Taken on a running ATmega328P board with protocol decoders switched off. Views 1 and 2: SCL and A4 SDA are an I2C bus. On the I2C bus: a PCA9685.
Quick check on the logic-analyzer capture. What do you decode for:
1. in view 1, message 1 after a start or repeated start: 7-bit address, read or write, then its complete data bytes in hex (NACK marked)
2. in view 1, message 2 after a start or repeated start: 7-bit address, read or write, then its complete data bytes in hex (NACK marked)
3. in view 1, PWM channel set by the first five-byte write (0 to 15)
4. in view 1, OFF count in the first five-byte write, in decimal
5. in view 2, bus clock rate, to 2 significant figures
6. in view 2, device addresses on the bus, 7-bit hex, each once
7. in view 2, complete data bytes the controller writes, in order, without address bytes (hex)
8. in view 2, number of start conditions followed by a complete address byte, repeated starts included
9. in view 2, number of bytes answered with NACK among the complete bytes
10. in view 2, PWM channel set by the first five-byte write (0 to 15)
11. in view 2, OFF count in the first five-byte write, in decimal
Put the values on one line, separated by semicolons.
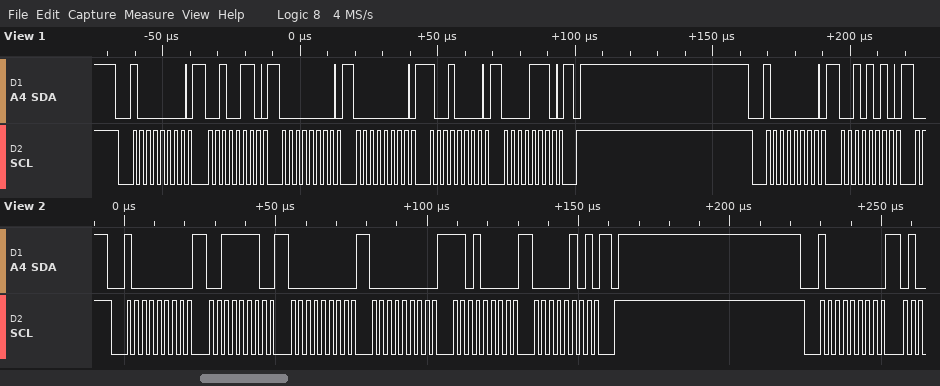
0x40 write: 26 00 00 90 0E; 0x40 write: 2A; 8; 3728; 400 kHz; 0x40; 3E 00 00 D0 05; 2; 0; 14; 1488
